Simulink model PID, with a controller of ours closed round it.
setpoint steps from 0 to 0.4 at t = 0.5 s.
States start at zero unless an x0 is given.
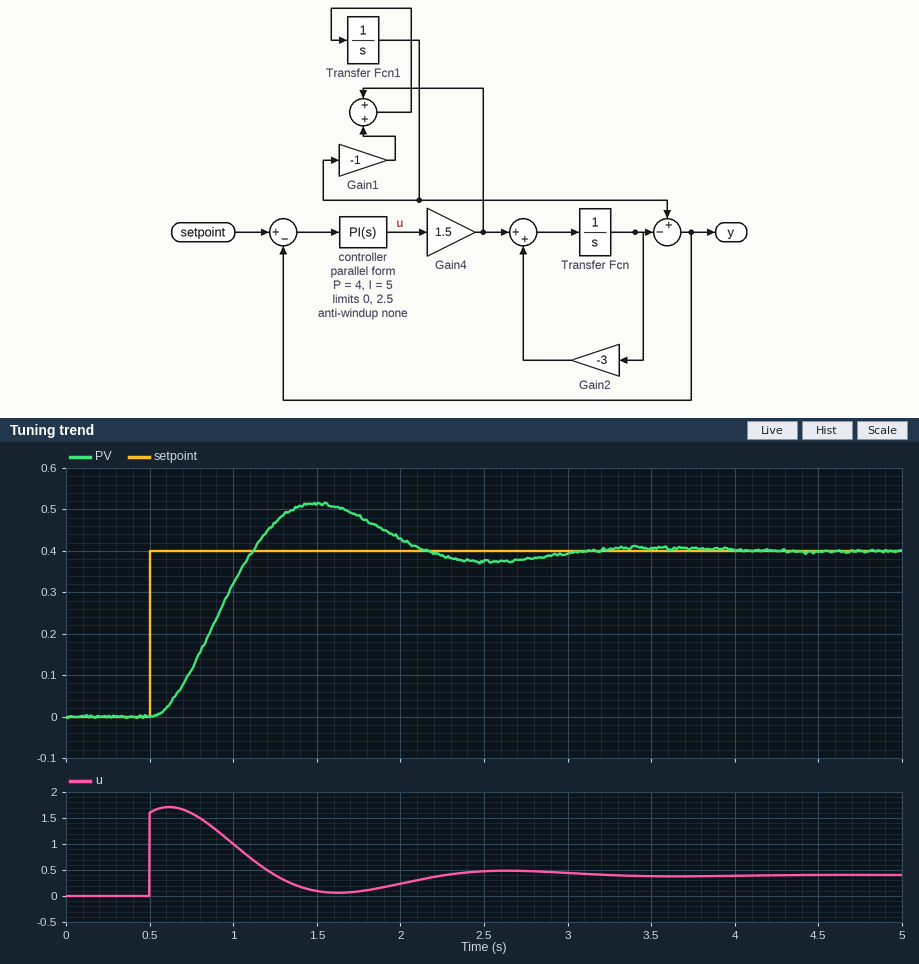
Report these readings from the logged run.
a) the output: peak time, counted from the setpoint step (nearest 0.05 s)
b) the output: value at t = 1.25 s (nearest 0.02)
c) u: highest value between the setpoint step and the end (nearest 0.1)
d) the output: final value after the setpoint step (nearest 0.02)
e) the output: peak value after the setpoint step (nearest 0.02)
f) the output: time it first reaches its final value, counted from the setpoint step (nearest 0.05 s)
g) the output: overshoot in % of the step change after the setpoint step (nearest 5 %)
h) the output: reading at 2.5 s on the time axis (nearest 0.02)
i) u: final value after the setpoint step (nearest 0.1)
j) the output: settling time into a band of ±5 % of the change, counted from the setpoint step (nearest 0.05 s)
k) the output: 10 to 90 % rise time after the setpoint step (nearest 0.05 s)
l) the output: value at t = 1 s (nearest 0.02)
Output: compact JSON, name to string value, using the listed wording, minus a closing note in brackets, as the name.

{"the output: peak time, counted from the setpoint step": "1.00 s", "the output: value at t = 1.25 s": "0.46", "u: highest value between the setpoint step and the end": "1.7", "the output: final value after the setpoint step": "0.40", "the output: peak value after the setpoint step": "0.52", "the output: time it first reaches its final value, counted from the setpoint step": "0.60 s", "the output: overshoot in % of the step change after the setpoint step": "30 %", "the output: reading at 2.5 s on the time axis": "0.38", "u: final value after the setpoint step": "0.4", "the output: settling time into a band of ±5 % of the change, counted from the setpoint step": "2.25 s", "the output: 10 to 90 % rise time after the setpoint step": "0.40 s", "the output: value at t = 1 s": "0.32"}
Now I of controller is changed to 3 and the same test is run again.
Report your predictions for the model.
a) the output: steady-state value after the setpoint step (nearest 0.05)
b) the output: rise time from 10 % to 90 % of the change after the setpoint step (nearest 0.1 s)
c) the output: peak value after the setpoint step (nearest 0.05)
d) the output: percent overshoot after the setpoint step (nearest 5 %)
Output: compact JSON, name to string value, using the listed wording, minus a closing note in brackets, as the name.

{"the output: steady-state value after the setpoint step": "0.40", "the output: rise time from 10 % to 90 % of the change after the setpoint step": "0.5 s", "the output: peak value after the setpoint step": "0.45", "the output: percent overshoot after the setpoint step": "15 %"}
